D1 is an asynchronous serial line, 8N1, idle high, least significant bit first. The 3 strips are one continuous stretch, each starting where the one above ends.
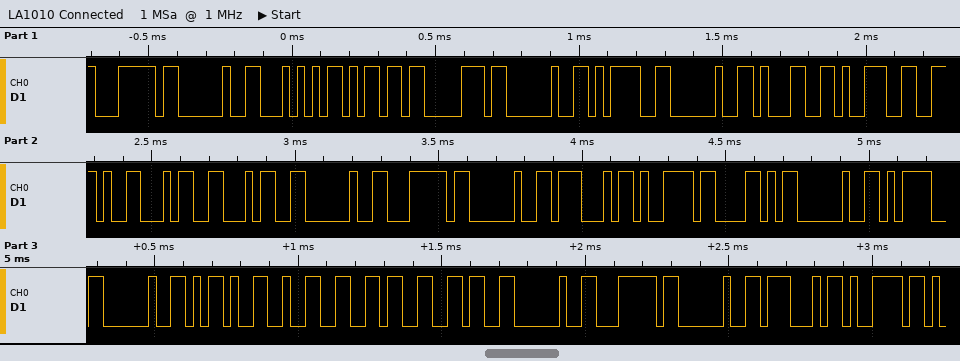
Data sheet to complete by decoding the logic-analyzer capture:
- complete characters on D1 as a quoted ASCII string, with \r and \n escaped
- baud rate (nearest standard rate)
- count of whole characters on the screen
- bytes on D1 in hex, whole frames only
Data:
"| Tmp = 19.44 | GyX = -266 | Gy"
38400 baud
31
0x7C 0x20 0x54 0x6D 0x70 0x20 0x3D 0x20 0x31 0x39 0x2E 0x34 0x34 0x20 0x7C 0x20 0x47 0x79 0x58 0x20 0x3D 0x20 0x2D 0x32 0x36 0x36 0x20 0x7C 0x20 0x47 0x79
